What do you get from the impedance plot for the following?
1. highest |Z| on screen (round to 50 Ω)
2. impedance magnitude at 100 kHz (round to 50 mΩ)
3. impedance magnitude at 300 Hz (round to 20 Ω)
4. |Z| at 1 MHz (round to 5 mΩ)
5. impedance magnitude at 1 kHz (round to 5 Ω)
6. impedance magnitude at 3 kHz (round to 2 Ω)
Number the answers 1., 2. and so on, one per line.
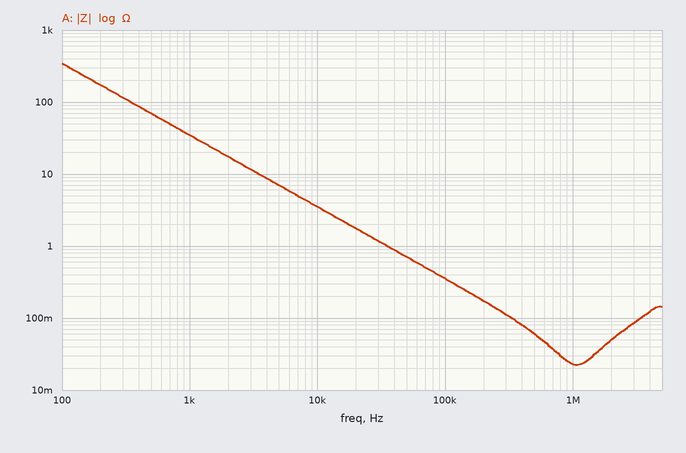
1. 350 Ω
2. 350 mΩ
3. 120 Ω
4. 25 mΩ
5. 35 Ω
6. 12 Ω
